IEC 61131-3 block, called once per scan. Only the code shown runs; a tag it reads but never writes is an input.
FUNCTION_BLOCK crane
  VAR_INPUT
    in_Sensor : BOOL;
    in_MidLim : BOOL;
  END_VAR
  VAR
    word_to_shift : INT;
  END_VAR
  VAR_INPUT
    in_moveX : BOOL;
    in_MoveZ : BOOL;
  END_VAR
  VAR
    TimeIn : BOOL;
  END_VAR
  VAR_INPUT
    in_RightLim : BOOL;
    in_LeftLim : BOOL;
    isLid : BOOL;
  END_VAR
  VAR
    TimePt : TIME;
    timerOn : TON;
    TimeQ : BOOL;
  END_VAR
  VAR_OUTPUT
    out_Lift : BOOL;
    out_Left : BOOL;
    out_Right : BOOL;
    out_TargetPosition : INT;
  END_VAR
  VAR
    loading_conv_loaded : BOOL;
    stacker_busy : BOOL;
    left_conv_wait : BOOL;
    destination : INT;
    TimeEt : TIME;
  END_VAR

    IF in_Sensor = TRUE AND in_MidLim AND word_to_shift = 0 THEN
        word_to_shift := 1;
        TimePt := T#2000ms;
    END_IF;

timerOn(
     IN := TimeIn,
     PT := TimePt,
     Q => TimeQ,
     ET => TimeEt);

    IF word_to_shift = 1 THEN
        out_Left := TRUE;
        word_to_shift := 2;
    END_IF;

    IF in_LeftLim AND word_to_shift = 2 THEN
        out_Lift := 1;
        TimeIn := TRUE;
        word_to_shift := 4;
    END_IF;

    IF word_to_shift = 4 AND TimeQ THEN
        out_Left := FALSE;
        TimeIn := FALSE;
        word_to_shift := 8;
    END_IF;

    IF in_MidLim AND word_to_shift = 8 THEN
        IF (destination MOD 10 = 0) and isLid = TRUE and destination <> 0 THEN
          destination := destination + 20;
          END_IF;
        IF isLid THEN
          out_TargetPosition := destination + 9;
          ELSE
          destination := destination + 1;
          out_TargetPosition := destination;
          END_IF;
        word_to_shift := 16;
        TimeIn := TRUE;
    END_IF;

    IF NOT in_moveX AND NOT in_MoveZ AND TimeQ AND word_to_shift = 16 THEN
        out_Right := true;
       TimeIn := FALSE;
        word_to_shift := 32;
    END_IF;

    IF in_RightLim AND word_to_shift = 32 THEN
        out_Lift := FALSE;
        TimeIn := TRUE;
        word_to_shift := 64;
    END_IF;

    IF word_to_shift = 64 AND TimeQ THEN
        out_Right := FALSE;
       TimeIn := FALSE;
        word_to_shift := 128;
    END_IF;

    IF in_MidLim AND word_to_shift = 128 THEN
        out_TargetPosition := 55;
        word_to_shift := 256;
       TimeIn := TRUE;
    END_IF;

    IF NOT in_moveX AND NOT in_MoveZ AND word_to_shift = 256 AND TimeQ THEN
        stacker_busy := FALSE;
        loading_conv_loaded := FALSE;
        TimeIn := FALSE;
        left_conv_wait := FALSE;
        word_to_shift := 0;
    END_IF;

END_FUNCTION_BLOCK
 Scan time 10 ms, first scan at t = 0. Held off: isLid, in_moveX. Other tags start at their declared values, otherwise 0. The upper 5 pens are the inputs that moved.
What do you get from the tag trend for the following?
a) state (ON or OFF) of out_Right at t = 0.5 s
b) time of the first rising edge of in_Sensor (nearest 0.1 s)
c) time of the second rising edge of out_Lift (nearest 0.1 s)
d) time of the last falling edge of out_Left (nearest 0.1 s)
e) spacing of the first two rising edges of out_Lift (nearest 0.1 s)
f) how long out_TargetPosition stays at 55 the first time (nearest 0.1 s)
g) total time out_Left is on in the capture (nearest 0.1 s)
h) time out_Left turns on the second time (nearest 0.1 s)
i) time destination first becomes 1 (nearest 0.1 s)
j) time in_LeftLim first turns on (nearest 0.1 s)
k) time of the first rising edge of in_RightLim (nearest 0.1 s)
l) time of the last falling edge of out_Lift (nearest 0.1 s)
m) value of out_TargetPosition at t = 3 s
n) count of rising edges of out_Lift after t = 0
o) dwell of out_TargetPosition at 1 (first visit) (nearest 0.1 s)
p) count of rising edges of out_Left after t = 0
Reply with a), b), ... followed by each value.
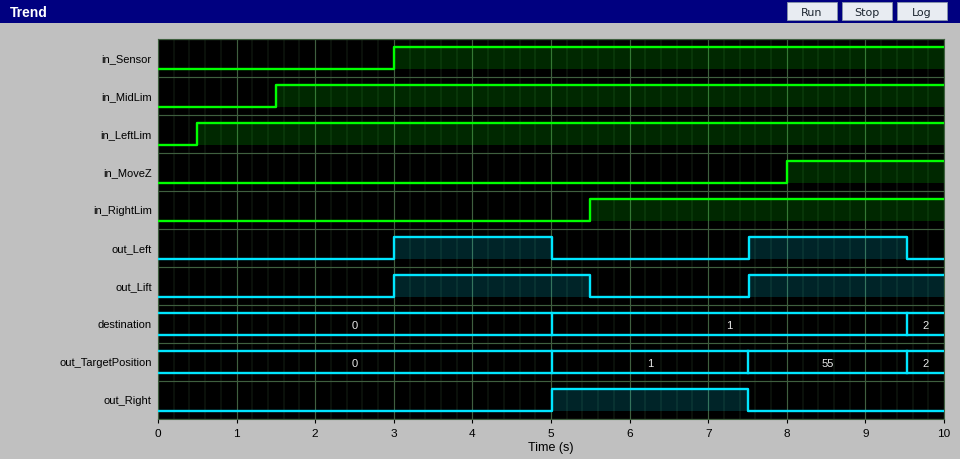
a) OFF
b) 3.0 s
c) 7.5 s
d) 9.5 s
e) 4.5 s
f) 2.0 s
g) 4.0 s
h) 7.5 s
i) 5.0 s
j) 0.5 s
k) 5.5 s
l) 5.5 s
m) 0
n) 2
o) 2.5 s
p) 2
